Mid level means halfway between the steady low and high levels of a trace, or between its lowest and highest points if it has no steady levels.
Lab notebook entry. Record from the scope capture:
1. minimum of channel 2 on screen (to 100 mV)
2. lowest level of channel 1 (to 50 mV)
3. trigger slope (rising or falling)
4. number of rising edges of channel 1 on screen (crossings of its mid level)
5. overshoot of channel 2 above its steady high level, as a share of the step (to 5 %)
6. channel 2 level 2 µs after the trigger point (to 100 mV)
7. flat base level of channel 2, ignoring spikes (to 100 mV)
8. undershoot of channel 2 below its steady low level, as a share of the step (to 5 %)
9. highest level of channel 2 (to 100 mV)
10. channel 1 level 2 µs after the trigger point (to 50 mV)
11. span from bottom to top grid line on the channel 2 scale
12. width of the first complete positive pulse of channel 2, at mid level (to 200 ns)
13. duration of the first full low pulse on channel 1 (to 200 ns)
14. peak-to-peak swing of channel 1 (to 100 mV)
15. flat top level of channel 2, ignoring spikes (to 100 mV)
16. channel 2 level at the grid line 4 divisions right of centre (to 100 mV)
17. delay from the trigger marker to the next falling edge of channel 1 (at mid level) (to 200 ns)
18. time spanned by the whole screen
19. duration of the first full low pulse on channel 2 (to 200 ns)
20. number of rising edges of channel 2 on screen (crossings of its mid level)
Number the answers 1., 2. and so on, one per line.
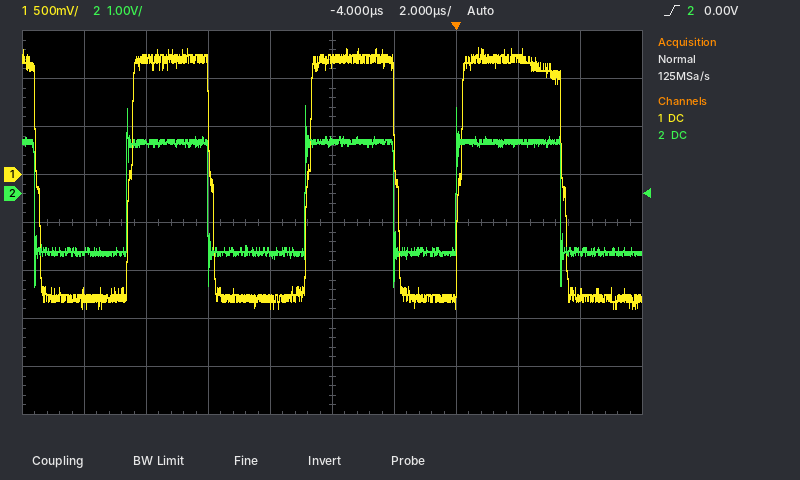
1. -1.9 V
2. -1.40 V
3. rising
4. 3
5. 30 %
6. 1.1 V
7. -1.2 V
8. 30 %
9. 1.8 V
10. 1.20 V
11. 8 V
12. 2.6 µs
13. 3.0 µs
14. 2.70 V
15. 1.1 V
16. -1.2 V
17. 3.4 µs
18. 20 µs
19. 3.0 µs
20. 3
